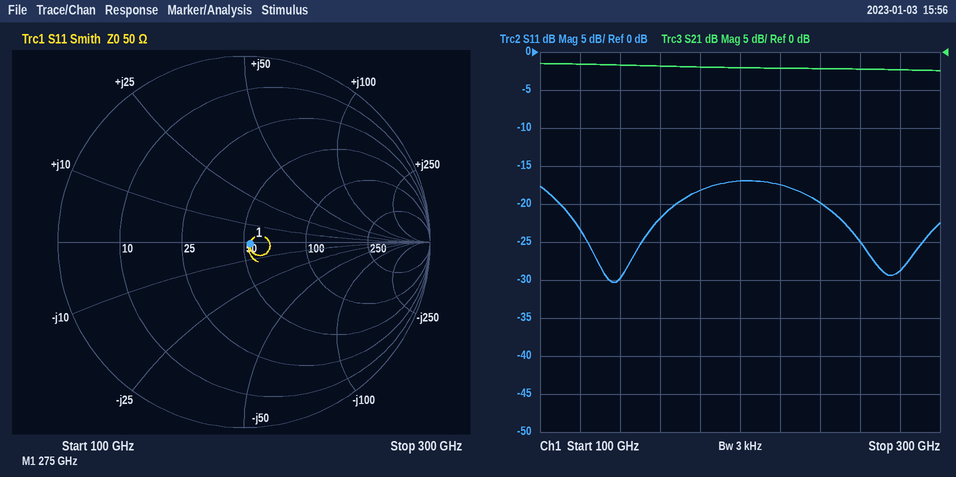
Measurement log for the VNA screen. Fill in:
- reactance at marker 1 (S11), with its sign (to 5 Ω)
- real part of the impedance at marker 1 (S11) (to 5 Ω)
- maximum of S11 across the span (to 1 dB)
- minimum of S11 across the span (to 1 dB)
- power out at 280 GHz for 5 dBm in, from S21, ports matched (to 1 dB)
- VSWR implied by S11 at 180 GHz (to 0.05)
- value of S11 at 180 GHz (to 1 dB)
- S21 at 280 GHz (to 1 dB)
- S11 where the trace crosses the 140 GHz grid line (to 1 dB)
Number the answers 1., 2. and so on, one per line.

1. 0 Ω
2. 55 Ω
3. -17 dB
4. -30 dB
5. 3 dBm
6. 1.30
7. -18 dB
8. -2 dB
9. -30 dB
